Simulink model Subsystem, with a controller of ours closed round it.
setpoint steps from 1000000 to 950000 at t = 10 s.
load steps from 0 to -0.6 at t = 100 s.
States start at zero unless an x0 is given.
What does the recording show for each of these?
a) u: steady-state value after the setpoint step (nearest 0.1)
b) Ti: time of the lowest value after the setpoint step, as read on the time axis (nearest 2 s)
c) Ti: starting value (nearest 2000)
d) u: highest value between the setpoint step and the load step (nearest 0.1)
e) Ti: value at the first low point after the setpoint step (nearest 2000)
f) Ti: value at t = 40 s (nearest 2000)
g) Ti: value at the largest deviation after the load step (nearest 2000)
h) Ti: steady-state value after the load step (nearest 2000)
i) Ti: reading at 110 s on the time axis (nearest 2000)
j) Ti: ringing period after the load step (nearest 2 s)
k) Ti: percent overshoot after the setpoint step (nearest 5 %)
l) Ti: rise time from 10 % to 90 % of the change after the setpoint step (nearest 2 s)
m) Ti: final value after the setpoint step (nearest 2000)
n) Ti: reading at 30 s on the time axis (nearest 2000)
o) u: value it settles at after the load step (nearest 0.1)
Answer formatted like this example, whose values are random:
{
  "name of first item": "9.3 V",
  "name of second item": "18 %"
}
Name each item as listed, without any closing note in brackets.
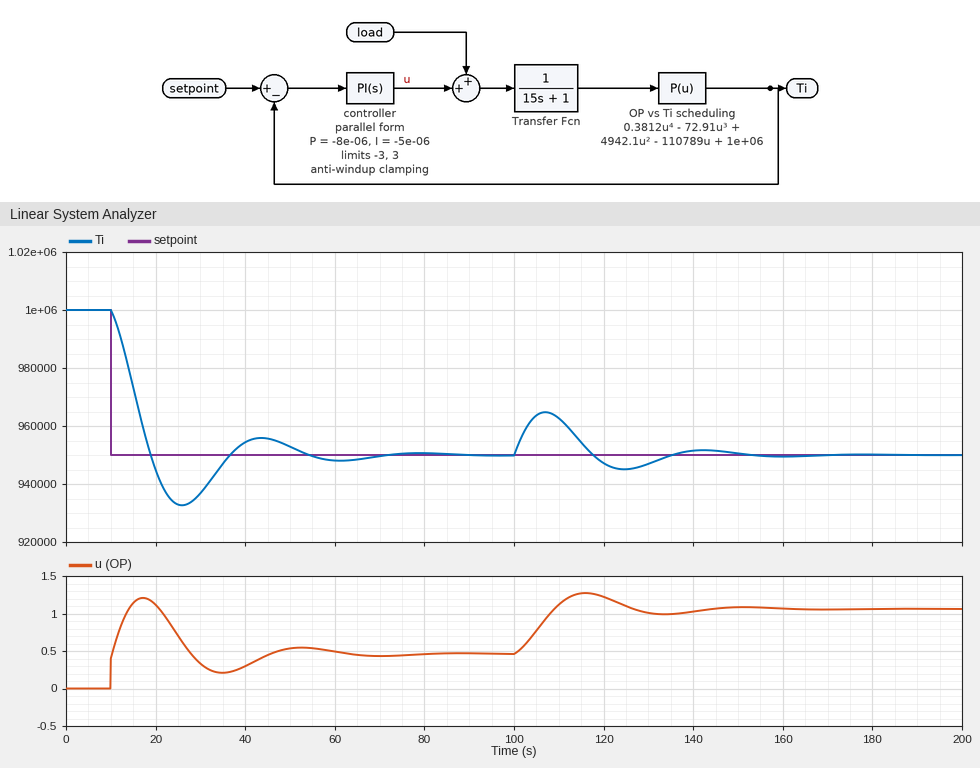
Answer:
{
  "u: steady-state value after the setpoint step": "0.5",
  "Ti: time of the lowest value after the setpoint step, as read on the time axis": "26 s",
  "Ti: starting value": "1000000",
  "u: highest value between the setpoint step and the load step": "1.2",
  "Ti: value at the first low point after the setpoint step": "932000",
  "Ti: value at t = 40 s": "954000",
  "Ti: value at the largest deviation after the load step": "964000",
  "Ti: steady-state value after the load step": "950000",
  "Ti: reading at 110 s on the time axis": "962000",
  "Ti: ringing period after the load step": "36 s",
  "Ti: percent overshoot after the setpoint step": "35 %",
  "Ti: rise time from 10 % to 90 % of the change after the setpoint step": "6 s",
  "Ti: final value after the setpoint step": "950000",
  "Ti: reading at 30 s on the time axis": "936000",
  "u: value it settles at after the load step": "1.1"
}
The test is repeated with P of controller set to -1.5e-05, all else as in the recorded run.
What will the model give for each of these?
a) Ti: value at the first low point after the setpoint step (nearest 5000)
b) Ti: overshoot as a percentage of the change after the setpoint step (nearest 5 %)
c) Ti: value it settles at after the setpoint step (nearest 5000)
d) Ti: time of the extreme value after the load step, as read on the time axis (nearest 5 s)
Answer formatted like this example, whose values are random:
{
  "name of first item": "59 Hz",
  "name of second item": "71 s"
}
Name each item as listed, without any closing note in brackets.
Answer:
{
  "Ti: value at the first low point after the setpoint step": "940000",
  "Ti: overshoot as a percentage of the change after the setpoint step": "25 %",
  "Ti: value it settles at after the setpoint step": "950000",
  "Ti: time of the extreme value after the load step, as read on the time axis": "105 s"
}
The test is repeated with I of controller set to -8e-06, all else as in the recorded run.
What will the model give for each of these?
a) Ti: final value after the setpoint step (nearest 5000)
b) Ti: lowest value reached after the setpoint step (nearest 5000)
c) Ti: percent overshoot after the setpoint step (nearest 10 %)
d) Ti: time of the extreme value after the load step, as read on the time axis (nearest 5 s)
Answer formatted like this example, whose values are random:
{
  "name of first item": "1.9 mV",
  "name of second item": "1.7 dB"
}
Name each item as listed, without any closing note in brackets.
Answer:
{
  "Ti: final value after the setpoint step": "950000",
  "Ti: lowest value reached after the setpoint step": "930000",
  "Ti: percent overshoot after the setpoint step": "40 %",
  "Ti: time of the extreme value after the load step, as read on the time axis": "105 s"
}
